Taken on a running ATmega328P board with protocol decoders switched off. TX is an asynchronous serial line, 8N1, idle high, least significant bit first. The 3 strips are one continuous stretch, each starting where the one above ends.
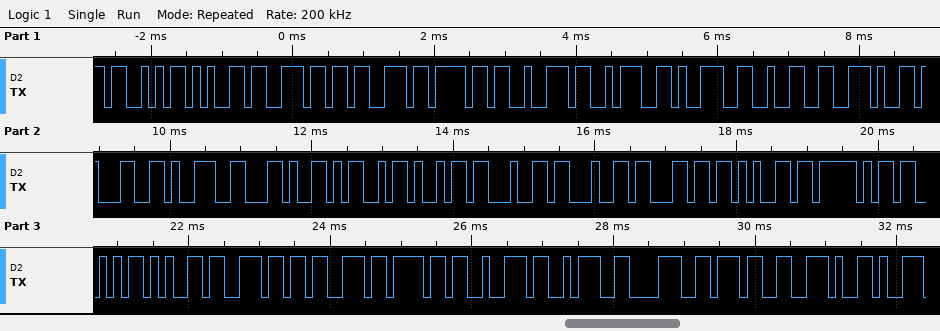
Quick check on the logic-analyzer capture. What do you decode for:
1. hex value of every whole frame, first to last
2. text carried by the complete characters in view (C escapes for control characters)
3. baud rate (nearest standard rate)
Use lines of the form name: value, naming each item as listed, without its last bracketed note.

hex value of every whole frame, first to last: 53 65 6E 73 6F 72 3A 39 32 2E 31 39 2C 4D 69 64 64 6C 65 5F 53 65 6E 73 6F 72 3A 38 37 2E
text carried by the complete characters in view: "Sensor:92.19,Middle_Sensor:87."
baud rate: 9600 baud
